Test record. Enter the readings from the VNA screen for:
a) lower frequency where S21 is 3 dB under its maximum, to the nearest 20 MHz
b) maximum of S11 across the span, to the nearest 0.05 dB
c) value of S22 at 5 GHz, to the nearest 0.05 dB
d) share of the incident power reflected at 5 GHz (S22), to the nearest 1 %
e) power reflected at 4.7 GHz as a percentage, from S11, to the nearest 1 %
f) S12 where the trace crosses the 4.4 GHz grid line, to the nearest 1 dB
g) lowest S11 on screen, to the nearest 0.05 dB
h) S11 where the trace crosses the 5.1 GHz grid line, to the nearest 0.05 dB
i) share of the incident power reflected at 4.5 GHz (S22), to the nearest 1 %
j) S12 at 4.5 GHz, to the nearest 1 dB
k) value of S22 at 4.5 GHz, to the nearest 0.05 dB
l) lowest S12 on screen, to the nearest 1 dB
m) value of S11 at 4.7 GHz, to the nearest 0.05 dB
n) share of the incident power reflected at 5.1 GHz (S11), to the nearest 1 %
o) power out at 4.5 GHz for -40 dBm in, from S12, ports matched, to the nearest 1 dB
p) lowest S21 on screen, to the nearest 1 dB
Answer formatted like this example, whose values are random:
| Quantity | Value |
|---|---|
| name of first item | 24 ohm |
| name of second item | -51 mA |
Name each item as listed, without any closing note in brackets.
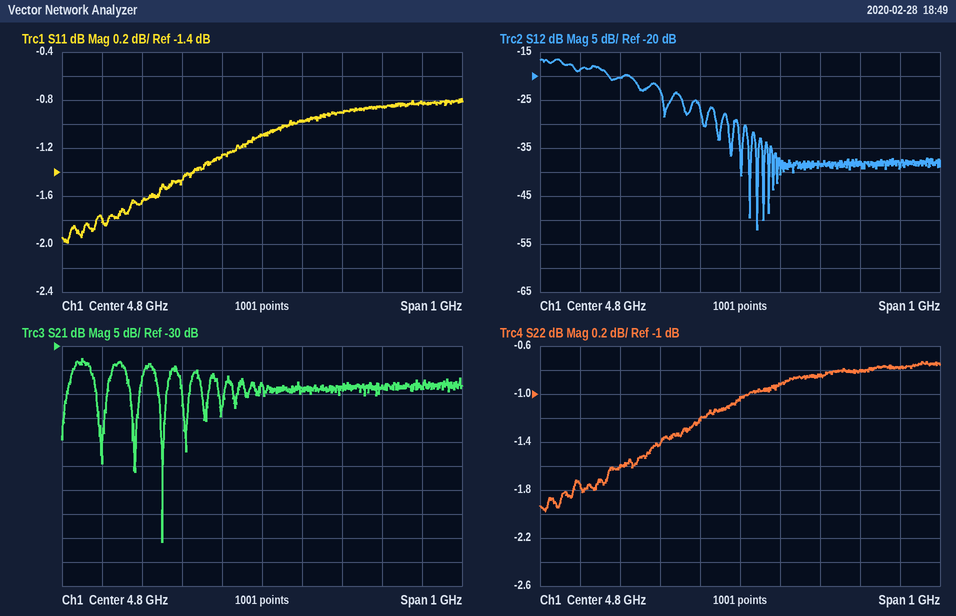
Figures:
| Quantity | Value |
|---|---|
| lower frequency where S21 is 3 dB under its maximum, to the nearest 20 MHz | 4.32 GHz |
| maximum of S11 across the span, to the nearest 0.05 dB | -0.80 dB |
| value of S22 at 5 GHz, to the nearest 0.05 dB | -0.85 dB |
| share of the incident power reflected at 5 GHz (S22), to the nearest 1 % | 82 % |
| power reflected at 4.7 GHz as a percentage, from S11, to the nearest 1 % | 75 % |
| S12 where the trace crosses the 4.4 GHz grid line, to the nearest 1 dB | -19 dB |
| lowest S11 on screen, to the nearest 0.05 dB | -2.00 dB |
| S11 where the trace crosses the 5.1 GHz grid line, to the nearest 0.05 dB | -0.85 dB |
| share of the incident power reflected at 4.5 GHz (S22), to the nearest 1 % | 69 % |
| S12 at 4.5 GHz, to the nearest 1 dB | -20 dB |
| value of S22 at 4.5 GHz, to the nearest 0.05 dB | -1.60 dB |
| lowest S12 on screen, to the nearest 1 dB | -52 dB |
| value of S11 at 4.7 GHz, to the nearest 0.05 dB | -1.25 dB |
| share of the incident power reflected at 5.1 GHz (S11), to the nearest 1 % | 82 % |
| power out at 4.5 GHz for -40 dBm in, from S12, ports matched, to the nearest 1 dB | -60 dBm |
| lowest S21 on screen, to the nearest 1 dB | -71 dB |
